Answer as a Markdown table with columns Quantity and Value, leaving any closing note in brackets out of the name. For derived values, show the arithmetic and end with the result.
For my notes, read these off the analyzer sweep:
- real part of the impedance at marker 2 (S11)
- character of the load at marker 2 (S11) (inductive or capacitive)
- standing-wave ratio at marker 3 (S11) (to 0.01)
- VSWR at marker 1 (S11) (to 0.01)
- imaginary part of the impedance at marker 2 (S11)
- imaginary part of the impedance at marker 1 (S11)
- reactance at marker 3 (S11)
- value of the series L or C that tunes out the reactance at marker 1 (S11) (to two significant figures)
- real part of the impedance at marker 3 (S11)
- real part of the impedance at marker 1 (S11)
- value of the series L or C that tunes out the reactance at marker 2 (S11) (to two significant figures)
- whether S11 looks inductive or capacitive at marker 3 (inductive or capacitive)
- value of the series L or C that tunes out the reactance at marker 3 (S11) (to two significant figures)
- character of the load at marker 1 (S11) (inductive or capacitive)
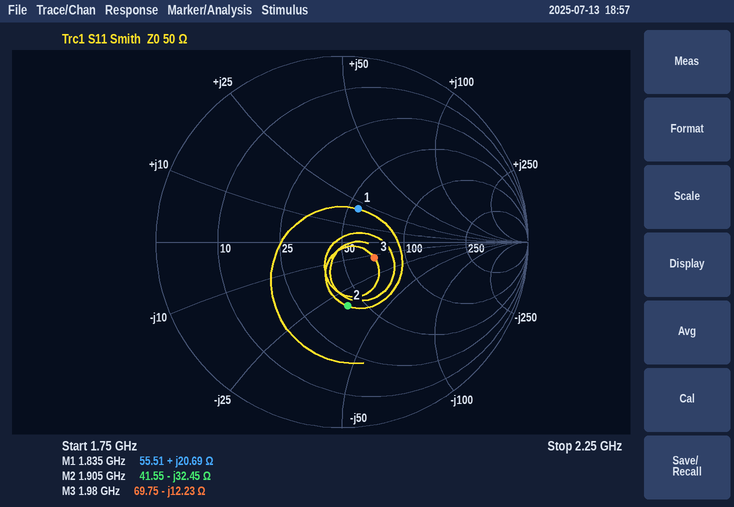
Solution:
| Quantity | Value |
|---|---|
| real part of the impedance at marker 2 | 41.55 Ω |
| character of the load at marker 2 (S11) | capacitive |
| standing-wave ratio at marker 3 (S11) | 1.48 |
| VSWR at marker 1 (S11) | 1.50 |
| imaginary part of the impedance at marker 2 | -32.45 Ω |
| imaginary part of the impedance at marker 1 | +20.69 Ω |
| reactance at marker 3 | -12.23 Ω |
| value of the series L or C that tunes out the reactance at marker 1 (S11) | C = 1/(2π × 1.835 GHz × 20.69 Ω) ≈ 4.2 pF |
| real part of the impedance at marker 3 | 69.75 Ω |
| real part of the impedance at marker 1 | 55.51 Ω |
| value of the series L or C that tunes out the reactance at marker 2 (S11) | L = 32.45 Ω/(2π × 1.905 GHz) ≈ 2.7 nH |
| whether S11 looks inductive or capacitive at marker 3 | capacitive |
| value of the series L or C that tunes out the reactance at marker 3 (S11) | L = 12.23 Ω/(2π × 1.98 GHz) ≈ 983 pH, so 980 pH to two significant figures |
| character of the load at marker 1 (S11) | inductive |
